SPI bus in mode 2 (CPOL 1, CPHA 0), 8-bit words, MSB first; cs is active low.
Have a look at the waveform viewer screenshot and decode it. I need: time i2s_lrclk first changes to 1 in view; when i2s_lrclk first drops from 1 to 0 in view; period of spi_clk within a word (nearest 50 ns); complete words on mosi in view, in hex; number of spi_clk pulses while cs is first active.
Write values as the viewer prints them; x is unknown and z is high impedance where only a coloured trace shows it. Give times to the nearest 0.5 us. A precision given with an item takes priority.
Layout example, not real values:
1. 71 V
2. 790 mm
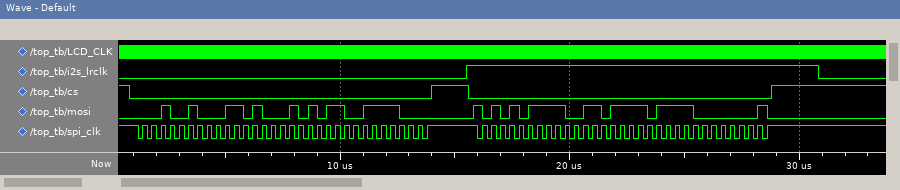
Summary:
1. 15.5 us
2. 31 us
3. 400 ns
4. 12, 34, 56, 78, AB, CD, EF, 01
5. 32
